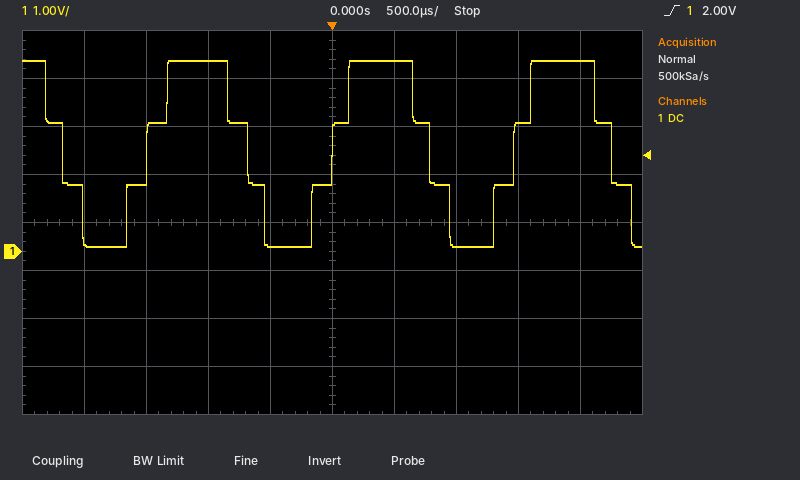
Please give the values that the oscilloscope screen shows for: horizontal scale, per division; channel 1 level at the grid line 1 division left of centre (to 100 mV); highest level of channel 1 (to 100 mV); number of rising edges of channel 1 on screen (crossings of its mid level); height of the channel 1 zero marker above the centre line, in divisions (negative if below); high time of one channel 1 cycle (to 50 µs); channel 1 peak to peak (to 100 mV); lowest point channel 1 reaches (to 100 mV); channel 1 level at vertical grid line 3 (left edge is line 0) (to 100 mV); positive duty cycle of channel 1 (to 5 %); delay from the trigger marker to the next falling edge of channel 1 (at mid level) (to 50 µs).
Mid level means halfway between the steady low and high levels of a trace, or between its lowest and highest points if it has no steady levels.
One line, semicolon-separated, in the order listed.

500 µs; 100 mV; 4.0 V; 3; -0.6 div; 800 µs; 3.9 V; 100 mV; 4.0 V; 55 %; 800 µs
